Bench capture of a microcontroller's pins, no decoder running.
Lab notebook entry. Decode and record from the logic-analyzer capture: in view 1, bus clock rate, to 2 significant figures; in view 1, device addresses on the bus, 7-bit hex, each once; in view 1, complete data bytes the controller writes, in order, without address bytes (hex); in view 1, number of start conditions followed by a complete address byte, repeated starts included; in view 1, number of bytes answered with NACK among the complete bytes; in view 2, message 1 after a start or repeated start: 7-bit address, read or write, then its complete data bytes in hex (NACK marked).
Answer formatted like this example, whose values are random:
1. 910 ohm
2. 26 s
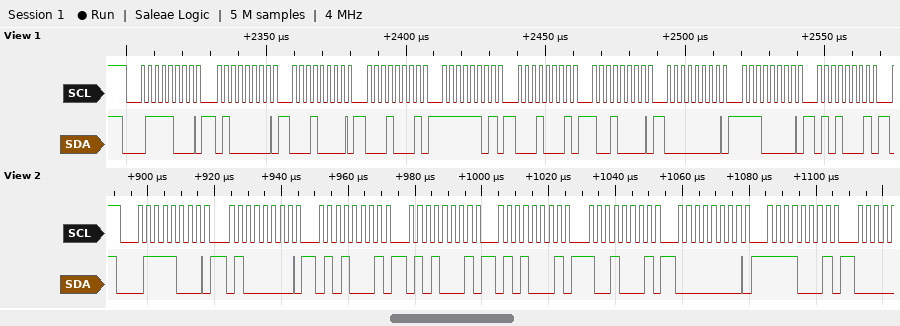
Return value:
1. 400 kHz
2. 0x3C
3. 40 10 11 FD 11 90 00 E0 51
4. 1
5. 0
6. 0x3C write: 40 51 51 51 91 00 F1
